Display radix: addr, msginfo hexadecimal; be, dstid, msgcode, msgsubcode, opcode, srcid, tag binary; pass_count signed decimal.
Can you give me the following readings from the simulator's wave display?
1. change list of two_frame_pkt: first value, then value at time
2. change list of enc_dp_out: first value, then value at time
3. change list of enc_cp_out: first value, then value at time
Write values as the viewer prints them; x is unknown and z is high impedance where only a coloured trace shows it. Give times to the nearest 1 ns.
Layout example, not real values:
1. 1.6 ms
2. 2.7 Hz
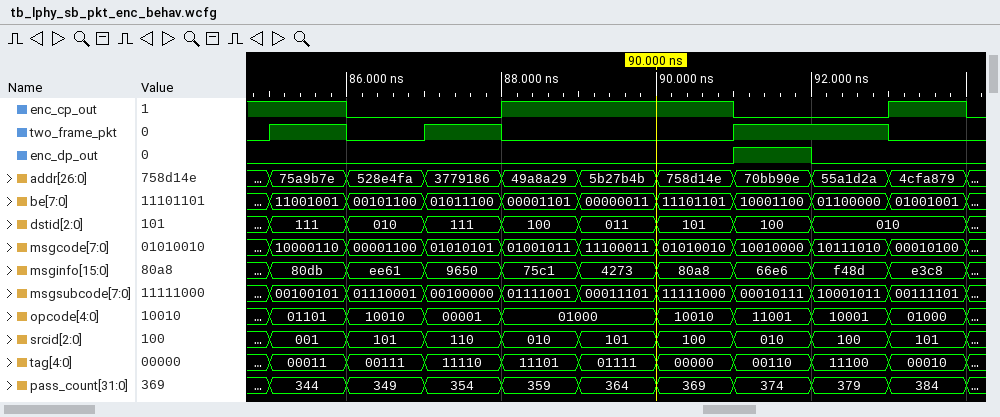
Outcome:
1. 0, 1 at 85 ns, 0 at 86 ns, 1 at 87 ns, 0 at 88 ns, 1 at 91 ns, 0 at 93 ns
2. 0, 1 at 91 ns, 0 at 92 ns
3. 1, 0 at 86 ns, 1 at 88 ns, 0 at 91 ns, 1 at 93 ns, 0 at 94 ns
